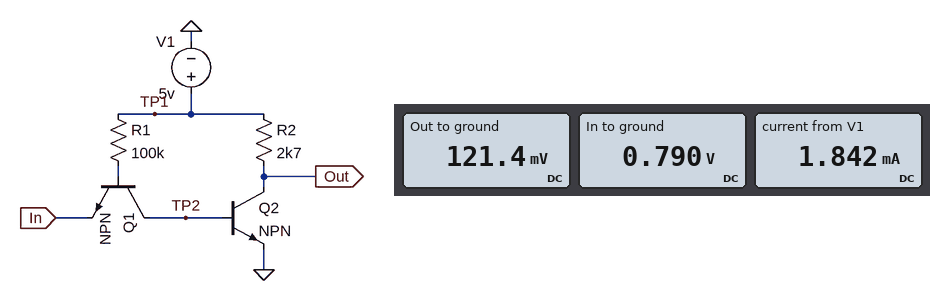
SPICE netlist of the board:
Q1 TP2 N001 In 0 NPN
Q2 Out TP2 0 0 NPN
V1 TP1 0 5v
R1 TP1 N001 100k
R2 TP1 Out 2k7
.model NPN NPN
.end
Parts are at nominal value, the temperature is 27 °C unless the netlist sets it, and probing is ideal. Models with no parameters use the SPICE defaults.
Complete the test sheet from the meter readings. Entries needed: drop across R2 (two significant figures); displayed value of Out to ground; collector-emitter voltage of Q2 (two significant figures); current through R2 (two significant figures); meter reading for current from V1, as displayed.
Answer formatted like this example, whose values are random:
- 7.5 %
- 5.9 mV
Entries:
- 4.9 V
- 121.4 mV
- 120 mV
- 1.8 mA
- 1.842 mA
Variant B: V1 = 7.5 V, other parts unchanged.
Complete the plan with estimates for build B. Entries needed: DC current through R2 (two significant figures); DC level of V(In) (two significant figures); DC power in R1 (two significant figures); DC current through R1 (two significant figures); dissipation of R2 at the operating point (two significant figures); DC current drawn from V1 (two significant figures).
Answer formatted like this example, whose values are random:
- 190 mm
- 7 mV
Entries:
- 2.7 mA
- 800 mV
- 360 µW
- 60 µA
- 20 mW
- 2.8 mA
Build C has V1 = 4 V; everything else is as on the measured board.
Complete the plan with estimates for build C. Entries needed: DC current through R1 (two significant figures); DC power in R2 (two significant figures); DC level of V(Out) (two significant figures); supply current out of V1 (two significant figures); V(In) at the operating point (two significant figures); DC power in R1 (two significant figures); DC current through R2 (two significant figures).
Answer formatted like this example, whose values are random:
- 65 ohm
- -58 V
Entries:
- 25 µA
- 5.6 mW
- 130 mV
- 1.5 mA
- 780 mV
- 64 µW
- 1.4 mA
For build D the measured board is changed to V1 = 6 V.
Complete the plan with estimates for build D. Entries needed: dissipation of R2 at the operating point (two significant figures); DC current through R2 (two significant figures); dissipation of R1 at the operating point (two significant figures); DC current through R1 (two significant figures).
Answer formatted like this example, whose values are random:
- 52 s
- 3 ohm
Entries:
- 13 mW
- 2.2 mA
- 200 µW
- 45 µA
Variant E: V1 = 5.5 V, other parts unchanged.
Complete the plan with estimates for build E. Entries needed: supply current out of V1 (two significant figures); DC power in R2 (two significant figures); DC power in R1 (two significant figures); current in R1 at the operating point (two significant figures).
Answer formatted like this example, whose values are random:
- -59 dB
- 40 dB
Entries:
- 2.0 mA
- 11 mW
- 160 µW
- 40 µA
